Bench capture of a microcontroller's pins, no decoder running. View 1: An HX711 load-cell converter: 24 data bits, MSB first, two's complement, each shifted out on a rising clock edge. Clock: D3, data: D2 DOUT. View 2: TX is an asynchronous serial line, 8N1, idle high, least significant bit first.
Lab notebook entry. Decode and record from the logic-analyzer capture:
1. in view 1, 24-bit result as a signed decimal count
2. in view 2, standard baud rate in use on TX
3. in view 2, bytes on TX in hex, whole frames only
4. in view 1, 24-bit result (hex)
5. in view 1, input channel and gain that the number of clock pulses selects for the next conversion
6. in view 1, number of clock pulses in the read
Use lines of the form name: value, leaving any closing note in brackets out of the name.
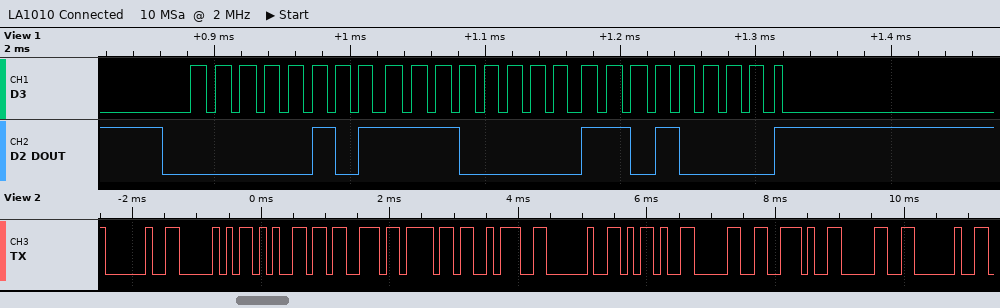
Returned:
in view 1, 24-bit result as a signed decimal count: 385232
in view 2, standard baud rate in use on TX: 9600 baud
in view 2, bytes on TX in hex, whole frames only: 20 50 65 73 6F 3A 20 2D 30 2E 30 20
in view 1, 24-bit result: 0x05E0D0
in view 1, input channel and gain that the number of clock pulses selects for the next conversion: channel A, gain 128
in view 1, number of clock pulses in the read: 25
